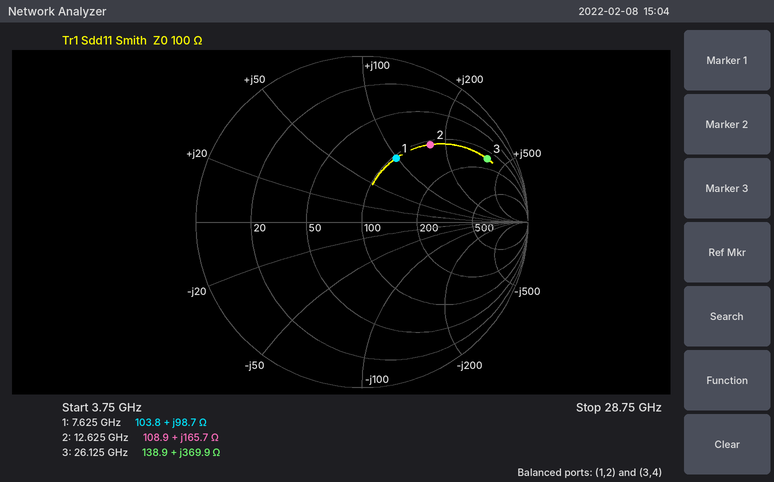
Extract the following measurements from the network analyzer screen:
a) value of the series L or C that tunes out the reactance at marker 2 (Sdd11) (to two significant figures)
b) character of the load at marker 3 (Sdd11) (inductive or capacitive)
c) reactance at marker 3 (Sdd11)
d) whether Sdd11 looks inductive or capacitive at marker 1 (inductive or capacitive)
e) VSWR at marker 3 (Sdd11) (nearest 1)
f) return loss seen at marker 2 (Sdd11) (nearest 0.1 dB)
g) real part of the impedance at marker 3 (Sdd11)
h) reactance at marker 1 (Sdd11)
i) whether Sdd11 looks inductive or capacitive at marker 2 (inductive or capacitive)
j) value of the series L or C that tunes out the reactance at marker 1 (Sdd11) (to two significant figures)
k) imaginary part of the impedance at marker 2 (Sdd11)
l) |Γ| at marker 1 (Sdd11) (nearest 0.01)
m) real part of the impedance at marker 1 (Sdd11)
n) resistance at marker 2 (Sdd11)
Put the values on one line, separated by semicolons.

76 fF; inductive; +369.9 Ω; inductive; 12; 4.1 dB; 138.9 Ω; +98.7 Ω; inductive; 210 fF; +165.7 Ω; 0.44; 103.8 Ω; 108.9 Ω
